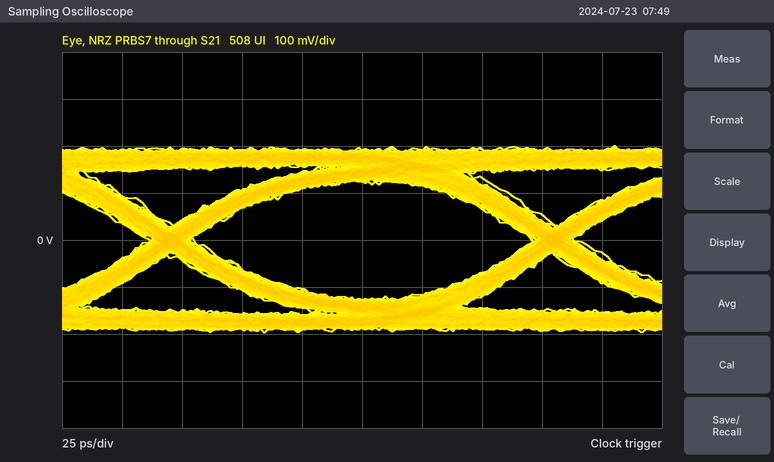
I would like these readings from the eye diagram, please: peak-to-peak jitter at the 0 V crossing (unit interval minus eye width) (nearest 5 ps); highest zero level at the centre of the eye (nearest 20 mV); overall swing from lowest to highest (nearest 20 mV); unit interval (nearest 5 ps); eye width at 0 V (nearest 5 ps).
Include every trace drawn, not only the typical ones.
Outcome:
20 ps
-120 mV
400 mV
160 ps
140 ps
